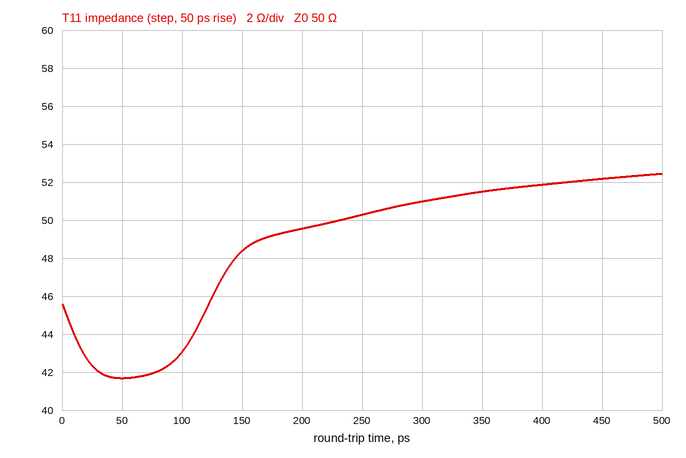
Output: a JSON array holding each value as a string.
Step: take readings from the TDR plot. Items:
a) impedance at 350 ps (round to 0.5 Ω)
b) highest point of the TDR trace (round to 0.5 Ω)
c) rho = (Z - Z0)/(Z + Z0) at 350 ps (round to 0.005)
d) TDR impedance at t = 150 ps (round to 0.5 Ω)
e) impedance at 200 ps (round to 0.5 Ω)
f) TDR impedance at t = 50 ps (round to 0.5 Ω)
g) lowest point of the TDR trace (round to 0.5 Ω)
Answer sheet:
["51.5 Ω", "52.5 Ω", "+0.015", "48.5 Ω", "49.5 Ω", "41.5 Ω", "41.5 Ω"]
